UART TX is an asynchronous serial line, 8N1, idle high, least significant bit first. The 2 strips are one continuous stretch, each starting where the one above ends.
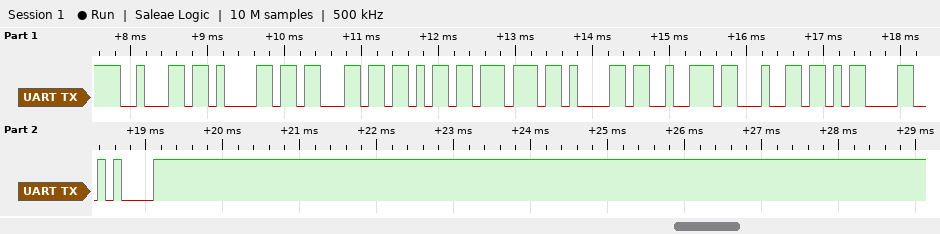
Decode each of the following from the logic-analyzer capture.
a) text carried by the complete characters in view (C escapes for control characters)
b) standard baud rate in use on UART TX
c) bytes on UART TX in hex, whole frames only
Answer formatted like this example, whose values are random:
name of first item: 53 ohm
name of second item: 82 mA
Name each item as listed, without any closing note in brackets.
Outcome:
text carried by the complete characters in view: "backward\r\n"
standard baud rate in use on UART TX: 9600 baud
bytes on UART TX in hex, whole frames only: 0x62 0x61 0x63 0x6B 0x77 0x61 0x72 0x64 0x0D 0x0A
